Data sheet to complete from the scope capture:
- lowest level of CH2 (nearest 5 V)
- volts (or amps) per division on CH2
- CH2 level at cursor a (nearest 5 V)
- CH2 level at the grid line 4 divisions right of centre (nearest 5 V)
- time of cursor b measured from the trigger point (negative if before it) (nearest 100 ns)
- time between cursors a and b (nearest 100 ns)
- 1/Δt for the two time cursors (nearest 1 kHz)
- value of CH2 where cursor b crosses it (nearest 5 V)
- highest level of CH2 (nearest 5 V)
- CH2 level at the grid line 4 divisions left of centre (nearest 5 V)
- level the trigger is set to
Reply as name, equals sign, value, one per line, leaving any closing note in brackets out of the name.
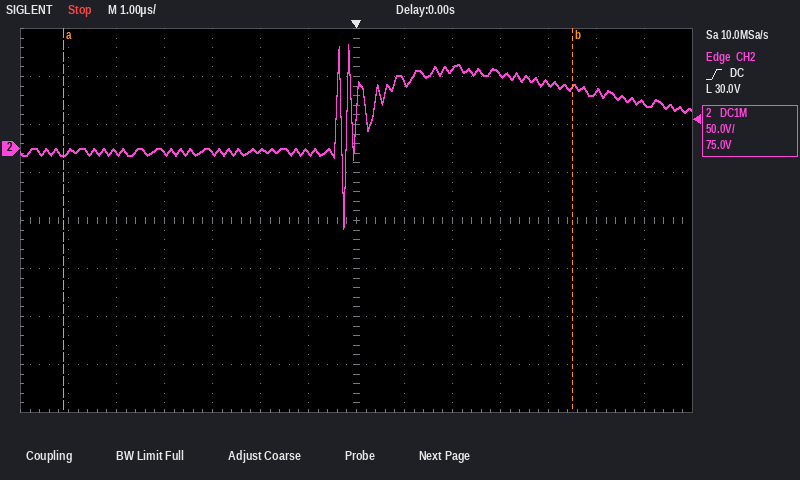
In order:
lowest level of CH2 = -85 V
volts (or amps) per division on CH2 = 50 V
CH2 level at cursor a = -5 V
CH2 level at the grid line 4 divisions right of centre = 70 V
time of cursor b measured from the trigger point (negative if before it) = +4.5 µs
time between cursors a and b = 10.6 µs
1/Δt for the two time cursors = 94 kHz
value of CH2 where cursor b crosses it = 65 V
highest level of CH2 = 110 V
CH2 level at the grid line 4 divisions left of centre = -5 V
level the trigger is set to = 30.0 V
